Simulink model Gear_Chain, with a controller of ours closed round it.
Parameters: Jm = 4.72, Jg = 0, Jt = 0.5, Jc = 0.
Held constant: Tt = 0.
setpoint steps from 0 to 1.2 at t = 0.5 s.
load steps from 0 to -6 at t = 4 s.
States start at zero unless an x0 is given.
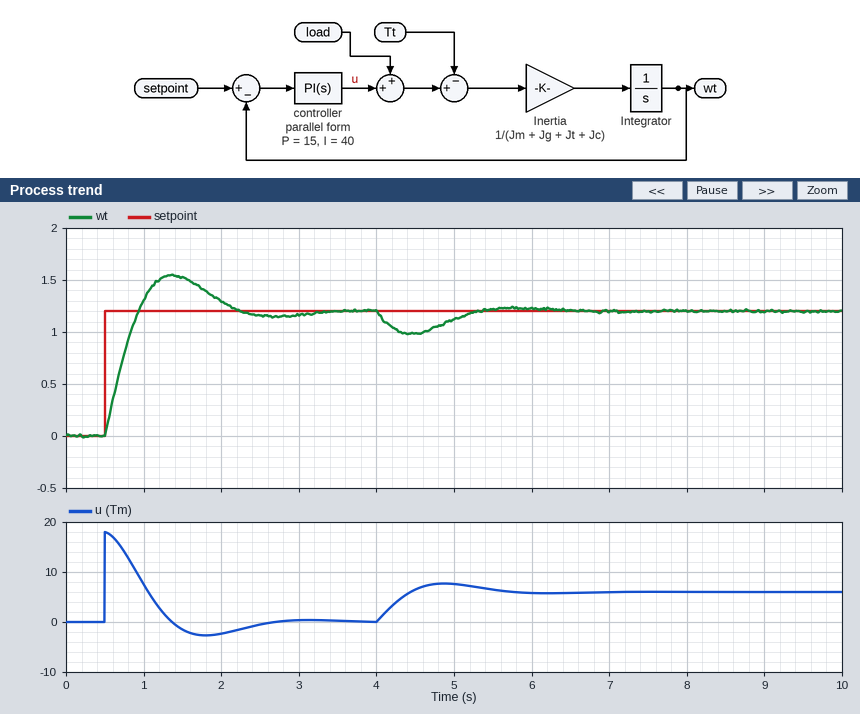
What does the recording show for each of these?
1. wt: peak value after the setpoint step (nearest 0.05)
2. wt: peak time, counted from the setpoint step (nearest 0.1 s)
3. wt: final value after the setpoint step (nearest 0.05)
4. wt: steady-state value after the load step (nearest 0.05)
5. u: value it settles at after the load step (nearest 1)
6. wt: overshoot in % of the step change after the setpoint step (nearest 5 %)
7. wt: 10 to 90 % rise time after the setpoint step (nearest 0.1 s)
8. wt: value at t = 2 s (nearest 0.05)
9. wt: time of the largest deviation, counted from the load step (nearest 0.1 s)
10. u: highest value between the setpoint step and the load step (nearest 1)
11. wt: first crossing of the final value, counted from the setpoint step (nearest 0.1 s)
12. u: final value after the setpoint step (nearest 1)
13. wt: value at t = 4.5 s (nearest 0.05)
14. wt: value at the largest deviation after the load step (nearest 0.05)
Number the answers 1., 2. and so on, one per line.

1. 1.55
2. 0.9 s
3. 1.20
4. 1.20
5. 6
6. 30 %
7. 0.3 s
8. 1.30
9. 0.4 s
10. 18
11. 0.4 s
12. 0
13. 1.00
14. 1.00
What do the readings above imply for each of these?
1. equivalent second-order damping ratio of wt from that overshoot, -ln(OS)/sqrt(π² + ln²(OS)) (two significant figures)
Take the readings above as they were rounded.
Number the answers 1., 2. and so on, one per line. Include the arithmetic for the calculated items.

1. ln(0.3) = -1.204; 1.204 / sqrt(9.870 + 1.450) = 0.36
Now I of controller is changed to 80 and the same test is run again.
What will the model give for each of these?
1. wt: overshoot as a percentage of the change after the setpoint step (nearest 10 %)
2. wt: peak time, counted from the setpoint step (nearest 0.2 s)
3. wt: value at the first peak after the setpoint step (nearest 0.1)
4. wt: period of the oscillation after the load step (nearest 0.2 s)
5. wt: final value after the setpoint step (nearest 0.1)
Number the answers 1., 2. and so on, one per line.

1. 40 %
2. 0.6 s
3. 1.7
4. 1.8 s
5. 1.2
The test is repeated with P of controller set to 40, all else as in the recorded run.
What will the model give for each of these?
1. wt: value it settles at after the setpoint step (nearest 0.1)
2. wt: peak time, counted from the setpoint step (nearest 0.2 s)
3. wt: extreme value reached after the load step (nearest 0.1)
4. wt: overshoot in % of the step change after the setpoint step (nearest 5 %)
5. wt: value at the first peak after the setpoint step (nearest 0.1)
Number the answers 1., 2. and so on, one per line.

1. 1.2
2. 0.6 s
3. 1.1
4. 10 %
5. 1.3
